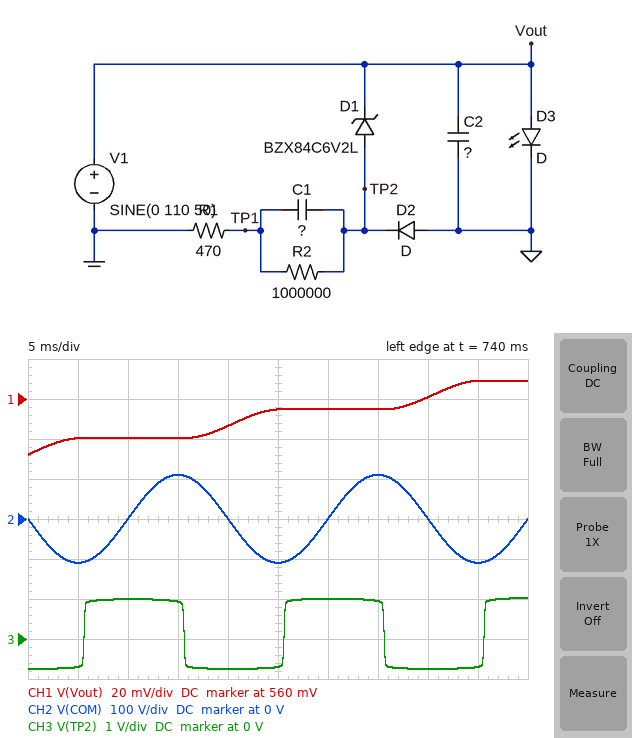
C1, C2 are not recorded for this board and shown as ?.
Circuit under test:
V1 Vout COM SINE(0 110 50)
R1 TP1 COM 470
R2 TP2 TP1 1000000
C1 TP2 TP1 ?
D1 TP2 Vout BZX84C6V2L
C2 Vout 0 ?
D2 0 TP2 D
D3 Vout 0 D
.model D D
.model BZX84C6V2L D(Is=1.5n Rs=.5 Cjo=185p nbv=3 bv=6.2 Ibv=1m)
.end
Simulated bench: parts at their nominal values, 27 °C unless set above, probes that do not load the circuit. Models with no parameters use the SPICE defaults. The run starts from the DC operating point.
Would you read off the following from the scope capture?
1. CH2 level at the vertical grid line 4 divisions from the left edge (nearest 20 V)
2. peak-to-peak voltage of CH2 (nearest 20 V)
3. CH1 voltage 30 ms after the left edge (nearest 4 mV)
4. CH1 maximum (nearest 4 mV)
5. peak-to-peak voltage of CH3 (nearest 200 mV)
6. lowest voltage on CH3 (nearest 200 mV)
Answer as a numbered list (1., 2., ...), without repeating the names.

1. 0 V
2. 220 V
3. 556 mV
4. 568 mV
5. 1.8 V
6. -800 mV
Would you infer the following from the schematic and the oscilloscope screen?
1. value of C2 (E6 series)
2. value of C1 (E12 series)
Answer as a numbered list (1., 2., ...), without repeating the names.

1. 15 mF
2. 1 µF
